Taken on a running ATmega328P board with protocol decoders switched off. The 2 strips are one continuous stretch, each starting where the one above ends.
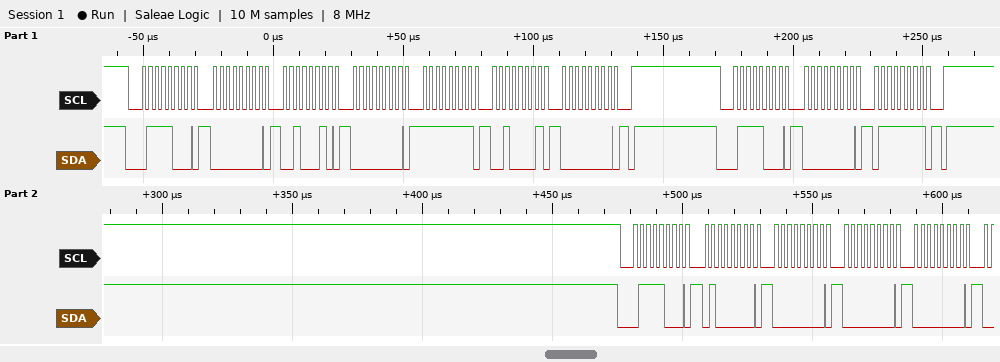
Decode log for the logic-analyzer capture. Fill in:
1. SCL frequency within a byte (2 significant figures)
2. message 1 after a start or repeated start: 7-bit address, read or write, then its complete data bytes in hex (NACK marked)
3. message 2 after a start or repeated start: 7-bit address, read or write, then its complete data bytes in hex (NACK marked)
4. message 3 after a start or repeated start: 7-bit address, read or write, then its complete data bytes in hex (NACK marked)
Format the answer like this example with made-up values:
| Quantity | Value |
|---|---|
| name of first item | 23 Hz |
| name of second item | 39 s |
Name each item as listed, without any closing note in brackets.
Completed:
| Quantity | Value |
|---|---|
| SCL frequency within a byte | 400 kHz |
| message 1 after a start or repeated start: 7-bit address, read or write, then its complete data bytes in hex | 0x3C write: 00 22 00 FF 21 00 |
| message 2 after a start or repeated start: 7-bit address, read or write, then its complete data bytes in hex | 0x3C write: 00 7F |
| message 3 after a start or repeated start: 7-bit address, read or write, then its complete data bytes in hex | 0x3C write: 40 00 00 00 |
